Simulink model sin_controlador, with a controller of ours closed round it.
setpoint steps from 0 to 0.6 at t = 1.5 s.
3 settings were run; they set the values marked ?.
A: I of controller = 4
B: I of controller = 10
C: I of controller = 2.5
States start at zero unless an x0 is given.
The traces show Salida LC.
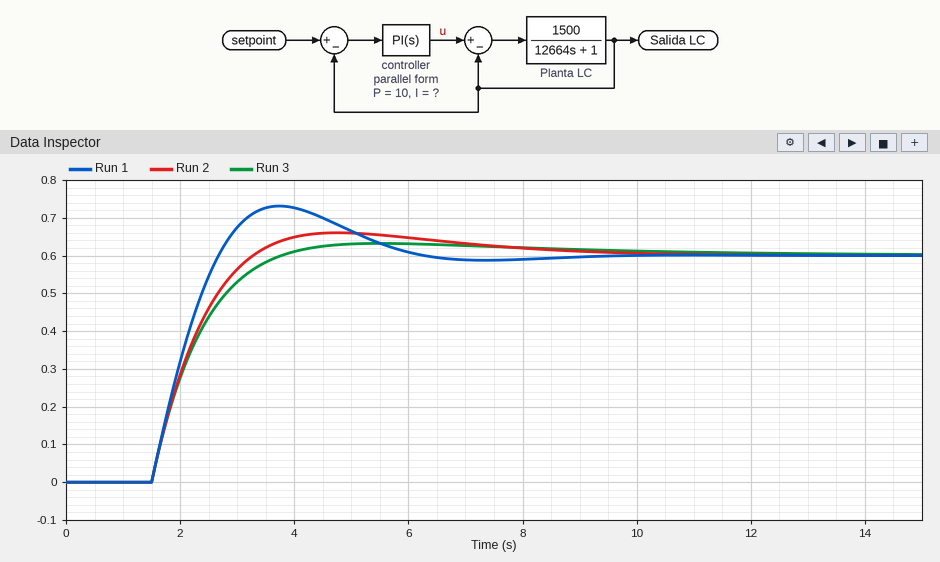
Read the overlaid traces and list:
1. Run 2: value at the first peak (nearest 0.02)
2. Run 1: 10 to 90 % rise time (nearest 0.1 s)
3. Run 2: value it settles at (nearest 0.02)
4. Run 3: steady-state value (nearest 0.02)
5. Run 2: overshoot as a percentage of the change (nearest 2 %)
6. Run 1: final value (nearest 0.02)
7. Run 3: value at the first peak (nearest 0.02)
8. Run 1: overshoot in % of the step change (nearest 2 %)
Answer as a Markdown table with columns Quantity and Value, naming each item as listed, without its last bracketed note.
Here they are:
| Quantity | Value |
|---|---|
| Run 2: value at the first peak | 0.66 |
| Run 1: 10 to 90 % rise time | 0.9 s |
| Run 2: value it settles at | 0.60 |
| Run 3: steady-state value | 0.60 |
| Run 2: overshoot as a percentage of the change | 10 % |
| Run 1: final value | 0.60 |
| Run 3: value at the first peak | 0.64 |
| Run 1: overshoot in % of the step change | 22 % |
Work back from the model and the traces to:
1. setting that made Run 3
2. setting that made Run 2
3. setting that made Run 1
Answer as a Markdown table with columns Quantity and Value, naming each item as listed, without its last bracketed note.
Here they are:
| Quantity | Value |
|---|---|
| setting that made Run 3 | C |
| setting that made Run 2 | A |
| setting that made Run 1 | B |
